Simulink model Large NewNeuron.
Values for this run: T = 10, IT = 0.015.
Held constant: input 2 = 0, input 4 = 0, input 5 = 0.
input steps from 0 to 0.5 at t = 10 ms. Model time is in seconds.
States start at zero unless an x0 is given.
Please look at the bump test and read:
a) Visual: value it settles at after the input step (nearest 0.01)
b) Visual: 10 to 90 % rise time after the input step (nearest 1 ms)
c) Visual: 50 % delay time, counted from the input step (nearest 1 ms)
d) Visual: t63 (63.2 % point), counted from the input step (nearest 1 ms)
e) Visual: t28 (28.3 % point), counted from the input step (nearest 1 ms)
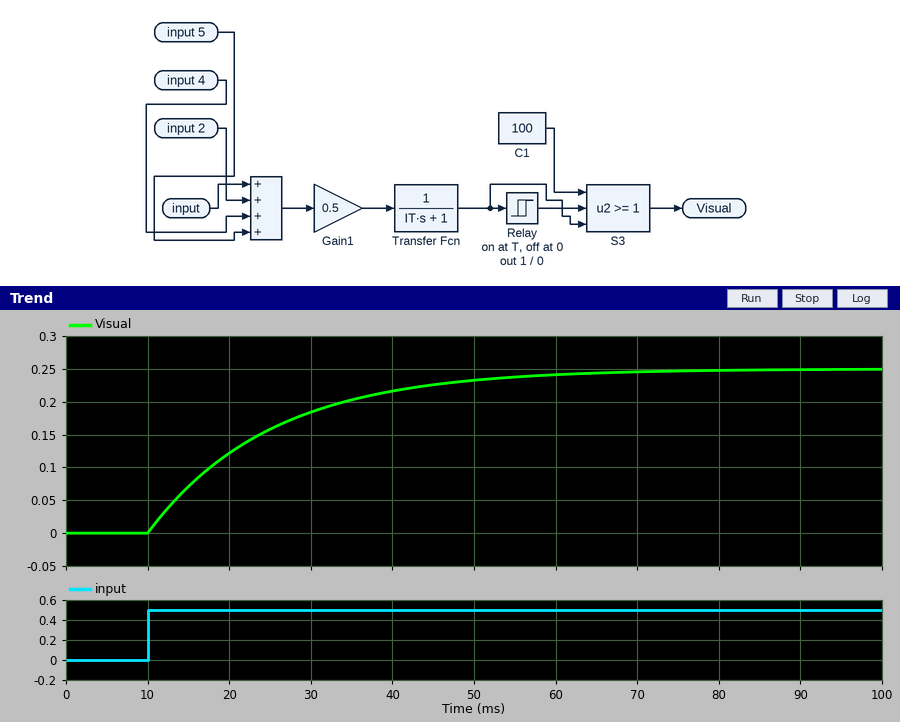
0.25
33 ms
10 ms
15 ms
5 ms
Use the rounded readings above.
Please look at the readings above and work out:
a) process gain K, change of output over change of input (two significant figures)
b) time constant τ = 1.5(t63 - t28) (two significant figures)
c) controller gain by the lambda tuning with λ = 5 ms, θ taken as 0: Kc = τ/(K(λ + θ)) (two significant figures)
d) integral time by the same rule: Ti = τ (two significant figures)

0.50
15 ms
6.0
15 ms
